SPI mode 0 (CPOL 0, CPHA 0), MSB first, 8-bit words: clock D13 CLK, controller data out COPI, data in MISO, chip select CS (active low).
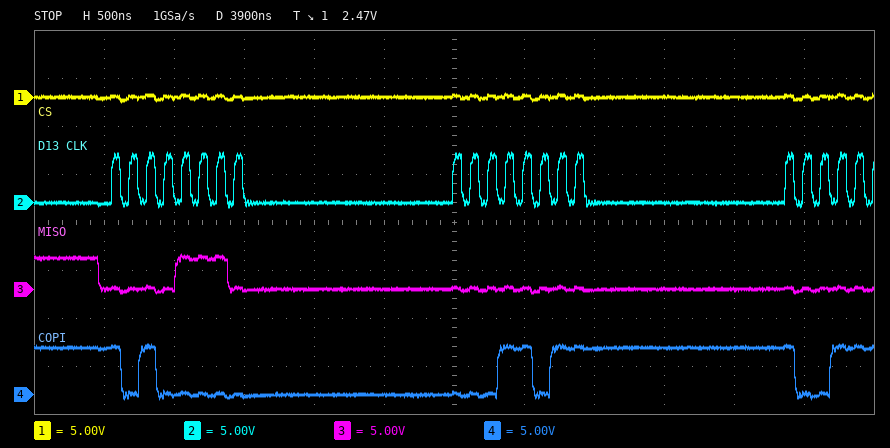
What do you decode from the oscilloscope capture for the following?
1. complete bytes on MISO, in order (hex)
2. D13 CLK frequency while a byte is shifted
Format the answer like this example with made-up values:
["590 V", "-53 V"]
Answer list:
["0E 00", "8 MHz"]
